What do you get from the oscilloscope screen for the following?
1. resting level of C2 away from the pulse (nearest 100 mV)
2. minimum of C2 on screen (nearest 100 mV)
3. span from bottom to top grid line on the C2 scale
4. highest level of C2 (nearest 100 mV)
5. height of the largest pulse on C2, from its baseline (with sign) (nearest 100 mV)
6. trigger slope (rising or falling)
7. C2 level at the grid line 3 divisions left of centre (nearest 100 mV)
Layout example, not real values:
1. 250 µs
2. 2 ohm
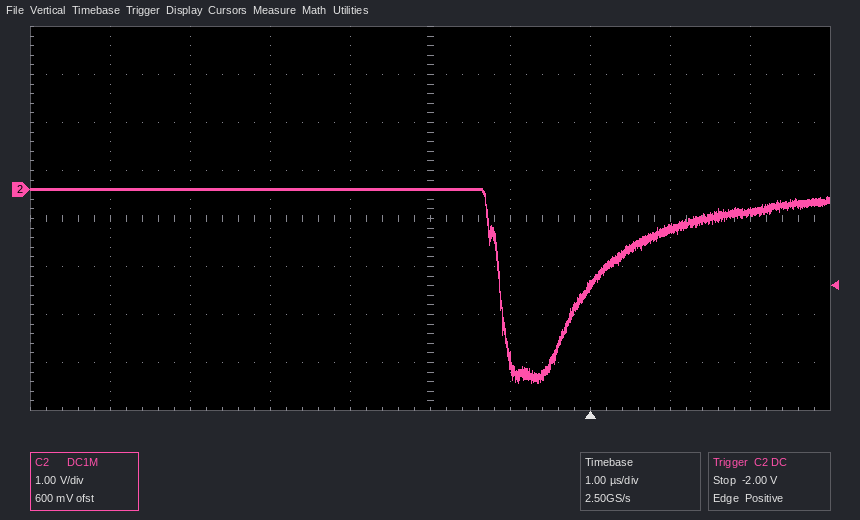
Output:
1. 0.0 V
2. -4.0 V
3. 8 V
4. 0.0 V
5. -4.0 V
6. rising
7. 0.0 V
